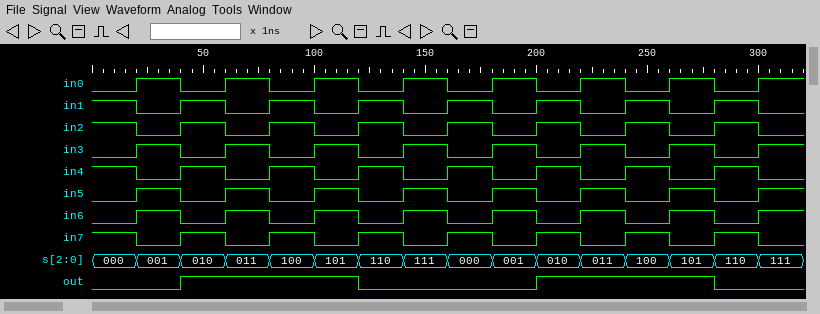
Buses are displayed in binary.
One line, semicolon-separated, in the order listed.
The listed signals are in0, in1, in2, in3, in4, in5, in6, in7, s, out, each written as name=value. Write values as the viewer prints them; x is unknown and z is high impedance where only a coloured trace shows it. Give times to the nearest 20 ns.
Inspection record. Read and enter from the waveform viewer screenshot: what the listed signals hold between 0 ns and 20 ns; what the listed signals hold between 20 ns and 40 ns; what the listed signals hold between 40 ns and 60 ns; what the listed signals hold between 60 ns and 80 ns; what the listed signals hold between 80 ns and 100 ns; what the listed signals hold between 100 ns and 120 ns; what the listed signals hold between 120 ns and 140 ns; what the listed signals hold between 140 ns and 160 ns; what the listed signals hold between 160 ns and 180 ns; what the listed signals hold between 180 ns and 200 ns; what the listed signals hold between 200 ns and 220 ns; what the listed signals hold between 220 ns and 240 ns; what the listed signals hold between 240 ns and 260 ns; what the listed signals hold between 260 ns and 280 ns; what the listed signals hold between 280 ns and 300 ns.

in0=0, in1=1, in2=1, in3=0, in4=1, in5=0, in6=0, in7=1, s=000, out=0; in0=1, in1=0, in2=0, in3=1, in4=0, in5=1, in6=1, in7=0, s=001, out=0; in0=0, in1=1, in2=1, in3=0, in4=1, in5=0, in6=0, in7=1, s=010, out=1; in0=1, in1=0, in2=0, in3=1, in4=0, in5=1, in6=1, in7=0, s=011, out=1; in0=0, in1=1, in2=1, in3=0, in4=1, in5=0, in6=0, in7=1, s=100, out=1; in0=1, in1=0, in2=0, in3=1, in4=0, in5=1, in6=1, in7=0, s=101, out=1; in0=0, in1=1, in2=1, in3=0, in4=1, in5=0, in6=0, in7=1, s=110, out=0; in0=1, in1=0, in2=0, in3=1, in4=0, in5=1, in6=1, in7=0, s=111, out=0; in0=0, in1=1, in2=1, in3=0, in4=1, in5=0, in6=0, in7=1, s=000, out=0; in0=1, in1=0, in2=0, in3=1, in4=0, in5=1, in6=1, in7=0, s=001, out=0; in0=0, in1=1, in2=1, in3=0, in4=1, in5=0, in6=0, in7=1, s=010, out=1; in0=1, in1=0, in2=0, in3=1, in4=0, in5=1, in6=1, in7=0, s=011, out=1; in0=0, in1=1, in2=1, in3=0, in4=1, in5=0, in6=0, in7=1, s=100, out=1; in0=1, in1=0, in2=0, in3=1, in4=0, in5=1, in6=1, in7=0, s=101, out=1; in0=0, in1=1, in2=1, in3=0, in4=1, in5=0, in6=0, in7=1, s=110, out=0
